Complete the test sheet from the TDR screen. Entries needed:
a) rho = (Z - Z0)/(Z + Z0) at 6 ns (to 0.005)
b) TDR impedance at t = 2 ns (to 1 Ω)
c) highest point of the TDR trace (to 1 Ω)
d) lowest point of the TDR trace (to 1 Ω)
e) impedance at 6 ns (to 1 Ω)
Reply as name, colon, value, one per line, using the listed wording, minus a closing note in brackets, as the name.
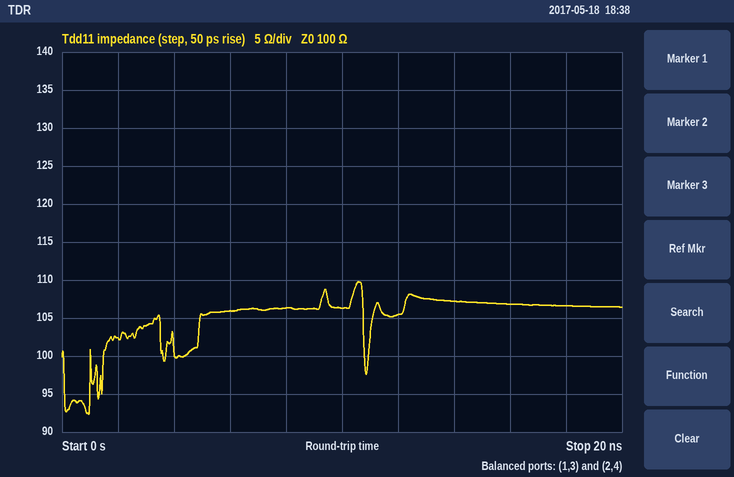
rho = (Z - Z0)/(Z + Z0) at 6 ns: +0.030
TDR impedance at t = 2 ns: 102 Ω
highest point of the TDR trace: 110 Ω
lowest point of the TDR trace: 92 Ω
impedance at 6 ns: 106 Ω
